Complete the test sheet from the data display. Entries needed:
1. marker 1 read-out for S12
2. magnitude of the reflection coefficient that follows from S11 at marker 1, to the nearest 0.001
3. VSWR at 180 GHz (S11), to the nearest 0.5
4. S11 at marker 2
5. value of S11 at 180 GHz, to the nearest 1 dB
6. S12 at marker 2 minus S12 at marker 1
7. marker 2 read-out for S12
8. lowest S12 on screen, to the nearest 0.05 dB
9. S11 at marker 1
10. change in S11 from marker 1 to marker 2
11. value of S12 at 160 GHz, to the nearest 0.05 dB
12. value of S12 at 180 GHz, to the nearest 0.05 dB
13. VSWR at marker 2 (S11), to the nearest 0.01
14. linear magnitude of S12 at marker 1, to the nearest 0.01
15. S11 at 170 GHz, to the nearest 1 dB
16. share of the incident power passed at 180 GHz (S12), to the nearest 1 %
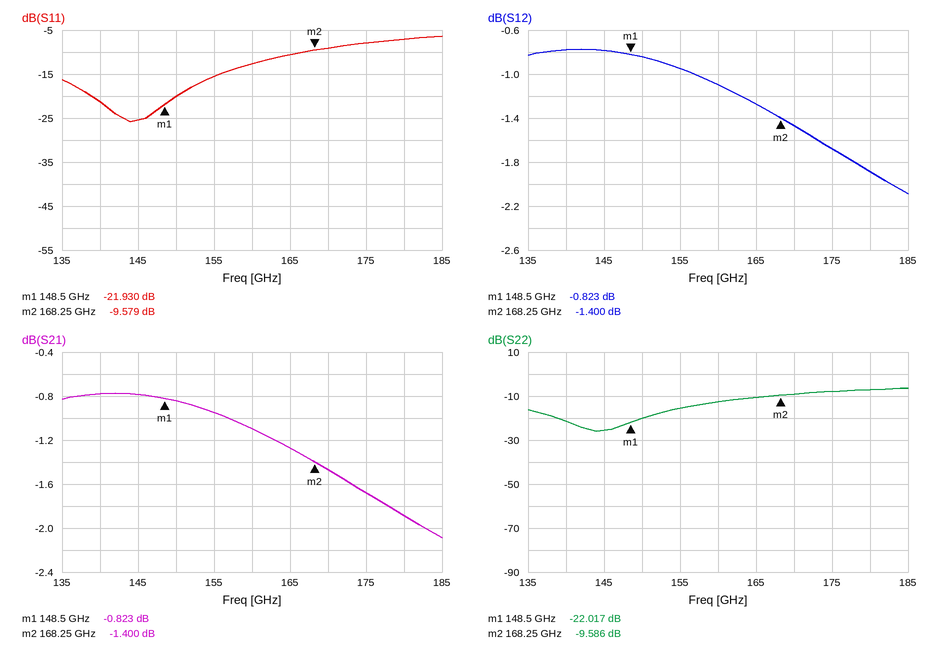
-0.823 dB
0.080
2.5
-9.579 dB
-7 dB
-0.577 dB
-1.400 dB
-2.10 dB
-21.930 dB
12.351 dB
-1.10 dB
-1.90 dB
1.99
0.91
-9 dB
65 %
